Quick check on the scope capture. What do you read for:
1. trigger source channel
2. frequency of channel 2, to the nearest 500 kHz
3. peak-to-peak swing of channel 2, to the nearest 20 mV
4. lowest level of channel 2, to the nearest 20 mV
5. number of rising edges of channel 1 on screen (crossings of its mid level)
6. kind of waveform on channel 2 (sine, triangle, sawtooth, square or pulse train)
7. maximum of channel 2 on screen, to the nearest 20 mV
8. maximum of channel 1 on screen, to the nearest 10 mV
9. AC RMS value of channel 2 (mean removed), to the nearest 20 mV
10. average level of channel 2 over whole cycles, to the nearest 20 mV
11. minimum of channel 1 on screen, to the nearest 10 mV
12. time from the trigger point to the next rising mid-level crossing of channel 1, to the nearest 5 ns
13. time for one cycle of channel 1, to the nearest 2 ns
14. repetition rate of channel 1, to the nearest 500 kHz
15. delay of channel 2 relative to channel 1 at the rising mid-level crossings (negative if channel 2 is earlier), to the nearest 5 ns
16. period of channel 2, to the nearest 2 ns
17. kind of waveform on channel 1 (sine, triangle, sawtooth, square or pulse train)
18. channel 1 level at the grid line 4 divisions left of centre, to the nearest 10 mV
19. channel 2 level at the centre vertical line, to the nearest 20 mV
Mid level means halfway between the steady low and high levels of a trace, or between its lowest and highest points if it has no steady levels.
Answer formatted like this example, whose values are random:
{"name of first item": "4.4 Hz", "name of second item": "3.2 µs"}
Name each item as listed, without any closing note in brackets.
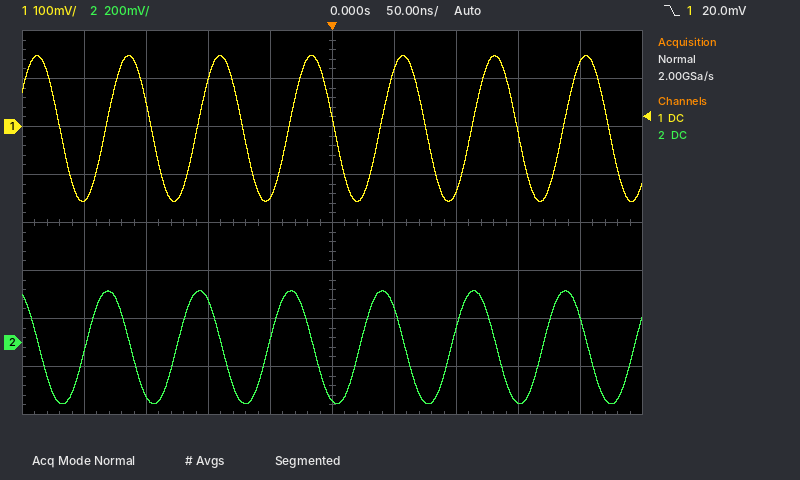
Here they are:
{"trigger source channel": "channel 1", "frequency of channel 2, to the nearest 500 kHz": "13.5 MHz", "peak-to-peak swing of channel 2, to the nearest 20 mV": "480 mV", "lowest level of channel 2, to the nearest 20 mV": "-260 mV", "number of rising edges of channel 1 on screen": "6", "kind of waveform on channel 2": "sine", "maximum of channel 2 on screen, to the nearest 20 mV": "220 mV", "maximum of channel 1 on screen, to the nearest 10 mV": "150 mV", "AC RMS value of channel 2 (mean removed), to the nearest 20 mV": "160 mV", "average level of channel 2 over whole cycles, to the nearest 20 mV": "-20 mV", "minimum of channel 1 on screen, to the nearest 10 mV": "-160 mV", "time from the trigger point to the next rising mid-level crossing of channel 1, to the nearest 5 ns": "40 ns", "time for one cycle of channel 1, to the nearest 2 ns": "74 ns", "repetition rate of channel 1, to the nearest 500 kHz": "13.5 MHz", "delay of channel 2 relative to channel 1 at the rising mid-level crossings (negative if channel 2 is earlier), to the nearest 5 ns": "-15 ns", "period of channel 2, to the nearest 2 ns": "74 ns", "kind of waveform on channel 1": "sine", "channel 1 level at the grid line 4 divisions left of centre, to the nearest 10 mV": "-150 mV", "channel 2 level at the centre vertical line, to the nearest 20 mV": "-240 mV"}
